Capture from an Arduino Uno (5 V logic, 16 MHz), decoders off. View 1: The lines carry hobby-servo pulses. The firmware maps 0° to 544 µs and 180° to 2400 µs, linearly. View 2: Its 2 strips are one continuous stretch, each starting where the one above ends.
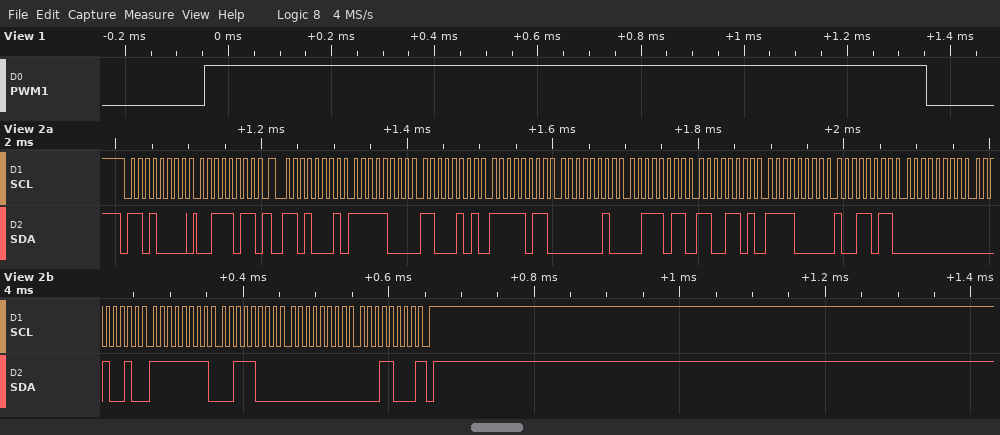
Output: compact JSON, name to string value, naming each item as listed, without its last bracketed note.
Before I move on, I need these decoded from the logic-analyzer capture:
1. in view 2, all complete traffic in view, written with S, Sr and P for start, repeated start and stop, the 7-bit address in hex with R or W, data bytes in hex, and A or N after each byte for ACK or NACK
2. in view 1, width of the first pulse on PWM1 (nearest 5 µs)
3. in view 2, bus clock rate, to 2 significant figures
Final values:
{"in view 2, all complete traffic in view, written with S, Sr and P for start, repeated start and stop, the 7-bit address in hex with R or W, data bytes in hex, and A or N after each byte for ACK or NACK": "S 68W A 3B A Sr 68R A F8 A C5 A FB A 02 A 3B A CD A F0 A 9B A 00 A 12 A FF A 38 A 00 A 18 N P", "in view 1, width of the first pulse on PWM1": "1400 µs", "in view 2, bus clock rate, to 2 significant figures": "100 kHz"}
